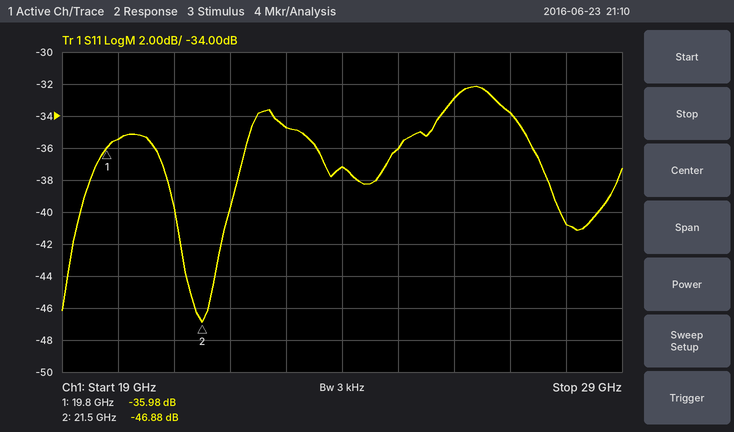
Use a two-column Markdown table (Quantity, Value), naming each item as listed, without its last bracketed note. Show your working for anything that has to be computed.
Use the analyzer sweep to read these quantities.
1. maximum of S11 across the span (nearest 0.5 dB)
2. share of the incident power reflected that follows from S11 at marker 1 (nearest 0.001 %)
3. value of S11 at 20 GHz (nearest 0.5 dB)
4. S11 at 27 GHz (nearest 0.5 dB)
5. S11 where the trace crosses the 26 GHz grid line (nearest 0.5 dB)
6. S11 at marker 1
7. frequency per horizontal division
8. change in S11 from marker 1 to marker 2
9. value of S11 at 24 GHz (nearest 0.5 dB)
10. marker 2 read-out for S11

| Quantity | Value |
|---|---|
| maximum of S11 across the span | -32.0 dB |
| share of the incident power reflected that follows from S11 at marker 1 | 10^(-35.98/10) ≈ 0.025 % |
| value of S11 at 20 GHz | -35.5 dB |
| S11 at 27 GHz | -34.0 dB |
| S11 where the trace crosses the 26 GHz grid line | -33.0 dB |
| S11 at marker 1 | -35.98 dB |
| frequency per horizontal division | 1 GHz |
| change in S11 from marker 1 to marker 2 | -46.88 − (-35.98) = -10.90 dB |
| value of S11 at 24 GHz | -37.0 dB |
| marker 2 read-out for S11 | -46.88 dB |
